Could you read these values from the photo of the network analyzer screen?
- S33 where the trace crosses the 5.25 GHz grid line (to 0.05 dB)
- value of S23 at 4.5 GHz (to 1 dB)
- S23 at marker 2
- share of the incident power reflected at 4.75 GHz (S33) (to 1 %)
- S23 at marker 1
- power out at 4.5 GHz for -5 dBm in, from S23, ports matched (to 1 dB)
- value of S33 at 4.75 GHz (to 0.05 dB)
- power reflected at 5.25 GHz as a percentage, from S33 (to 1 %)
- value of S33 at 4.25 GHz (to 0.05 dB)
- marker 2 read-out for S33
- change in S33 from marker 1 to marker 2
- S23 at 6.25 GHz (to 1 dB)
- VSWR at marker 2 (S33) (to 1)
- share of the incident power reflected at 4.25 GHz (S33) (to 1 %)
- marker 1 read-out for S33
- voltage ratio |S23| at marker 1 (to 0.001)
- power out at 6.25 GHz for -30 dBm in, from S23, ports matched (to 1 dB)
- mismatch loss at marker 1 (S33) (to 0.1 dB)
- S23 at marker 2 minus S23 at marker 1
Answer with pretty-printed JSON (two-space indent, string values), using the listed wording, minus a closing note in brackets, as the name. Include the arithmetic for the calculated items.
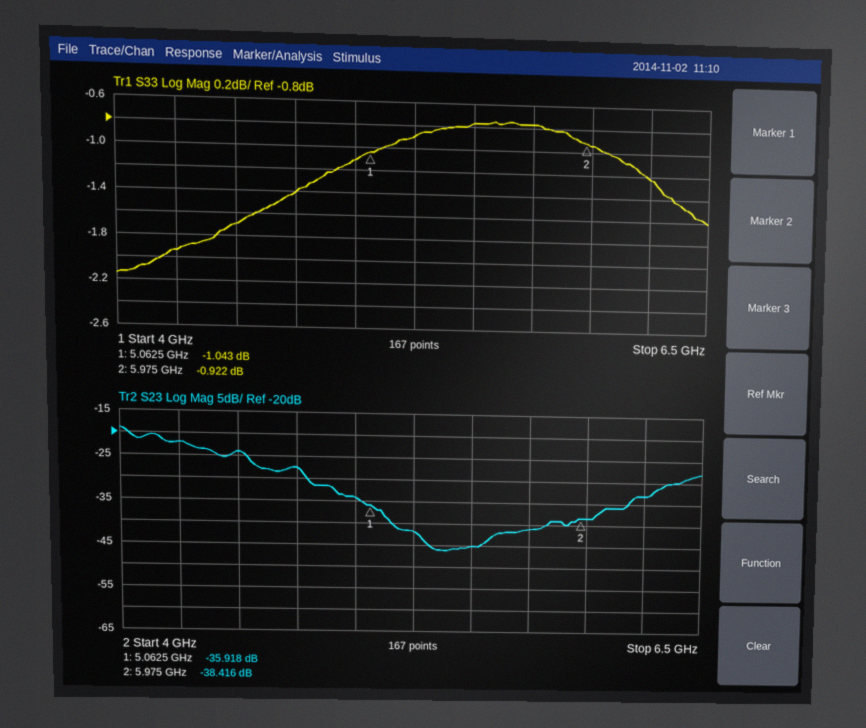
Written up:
{
  "S33 where the trace crosses the 5.25 GHz grid line": "-0.90 dB",
  "value of S23 at 4.5 GHz": "-24 dB",
  "S23 at marker 2": "-38.416 dB",
  "share of the incident power reflected at 4.75 GHz (S33)": "10^(-1.4/10) ≈ 72 %",
  "S23 at marker 1": "-35.918 dB",
  "power out at 4.5 GHz for -5 dBm in, from S23, ports matched": "-5 dBm + (-24 dB) = -29 dBm",
  "value of S33 at 4.75 GHz": "-1.40 dB",
  "power reflected at 5.25 GHz as a percentage, from S33": "10^(-0.9/10) ≈ 81 %",
  "value of S33 at 4.25 GHz": "-1.95 dB",
  "marker 2 read-out for S33": "-0.922 dB",
  "change in S33 from marker 1 to marker 2": "-0.922 − (-1.043) = 0.121 dB",
  "S23 at 6.25 GHz": "-33 dB",
  "VSWR at marker 2 (S33)": "(1 + 0.8993)/(1 − 0.8993) ≈ 19",
  "share of the incident power reflected at 4.25 GHz (S33)": "10^(-1.95/10) ≈ 64 %",
  "marker 1 read-out for S33": "-1.043 dB",
  "voltage ratio |S23| at marker 1": "10^(-35.918/20) ≈ 0.016",
  "power out at 6.25 GHz for -30 dBm in, from S23, ports matched": "-30 dBm + (-33 dB) = -63 dBm",
  "mismatch loss at marker 1 (S33)": "−10 log10(1 − 10^(-1.043/10)) ≈ 6.7 dB",
  "S23 at marker 2 minus S23 at marker 1": "-38.416 − (-35.918) = -2.498 dB"
}
